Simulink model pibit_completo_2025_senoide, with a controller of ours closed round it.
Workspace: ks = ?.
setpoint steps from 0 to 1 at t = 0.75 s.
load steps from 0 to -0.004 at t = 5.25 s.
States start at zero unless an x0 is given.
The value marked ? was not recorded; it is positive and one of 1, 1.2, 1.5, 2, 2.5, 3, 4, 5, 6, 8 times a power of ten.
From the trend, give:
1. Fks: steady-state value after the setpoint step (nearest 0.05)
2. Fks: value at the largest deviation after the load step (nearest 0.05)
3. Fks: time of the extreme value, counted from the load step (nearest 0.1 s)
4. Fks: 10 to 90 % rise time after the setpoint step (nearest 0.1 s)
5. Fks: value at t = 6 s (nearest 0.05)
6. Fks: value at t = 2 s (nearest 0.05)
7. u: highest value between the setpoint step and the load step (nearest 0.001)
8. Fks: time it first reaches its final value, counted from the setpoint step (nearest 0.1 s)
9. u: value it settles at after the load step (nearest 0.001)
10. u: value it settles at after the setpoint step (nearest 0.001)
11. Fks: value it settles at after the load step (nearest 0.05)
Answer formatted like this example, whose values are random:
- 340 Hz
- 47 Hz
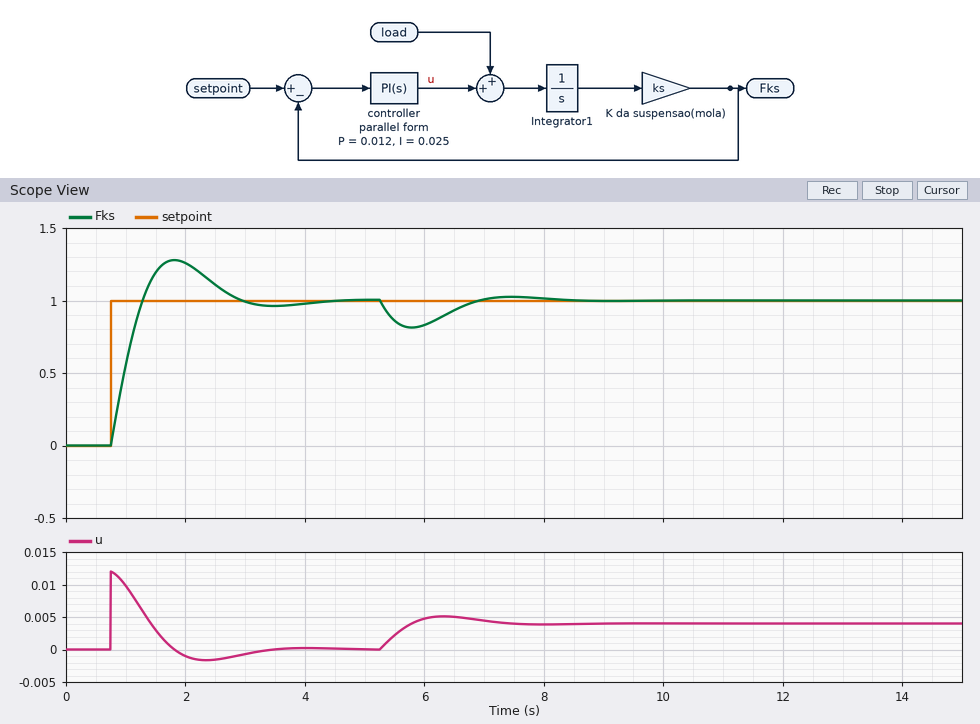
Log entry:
- 1.00
- 0.80
- 0.5 s
- 0.4 s
- 0.85
- 1.25
- 0.012
- 0.5 s
- 0.004
- 0.000
- 1.00
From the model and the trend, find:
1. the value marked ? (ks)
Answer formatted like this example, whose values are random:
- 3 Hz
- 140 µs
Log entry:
- 200
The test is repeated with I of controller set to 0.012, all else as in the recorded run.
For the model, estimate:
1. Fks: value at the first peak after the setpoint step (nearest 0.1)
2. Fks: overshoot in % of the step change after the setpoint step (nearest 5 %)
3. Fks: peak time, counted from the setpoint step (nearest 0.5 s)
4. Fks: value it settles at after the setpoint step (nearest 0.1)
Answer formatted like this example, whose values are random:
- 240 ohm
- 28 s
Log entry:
- 1.2
- 20 %
- 1.5 s
- 1.0
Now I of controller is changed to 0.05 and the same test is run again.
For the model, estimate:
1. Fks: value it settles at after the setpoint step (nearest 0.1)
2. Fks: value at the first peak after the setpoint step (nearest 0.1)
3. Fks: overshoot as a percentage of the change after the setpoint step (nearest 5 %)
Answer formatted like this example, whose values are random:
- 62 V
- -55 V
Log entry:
- 1.0
- 1.4
- 40 %
